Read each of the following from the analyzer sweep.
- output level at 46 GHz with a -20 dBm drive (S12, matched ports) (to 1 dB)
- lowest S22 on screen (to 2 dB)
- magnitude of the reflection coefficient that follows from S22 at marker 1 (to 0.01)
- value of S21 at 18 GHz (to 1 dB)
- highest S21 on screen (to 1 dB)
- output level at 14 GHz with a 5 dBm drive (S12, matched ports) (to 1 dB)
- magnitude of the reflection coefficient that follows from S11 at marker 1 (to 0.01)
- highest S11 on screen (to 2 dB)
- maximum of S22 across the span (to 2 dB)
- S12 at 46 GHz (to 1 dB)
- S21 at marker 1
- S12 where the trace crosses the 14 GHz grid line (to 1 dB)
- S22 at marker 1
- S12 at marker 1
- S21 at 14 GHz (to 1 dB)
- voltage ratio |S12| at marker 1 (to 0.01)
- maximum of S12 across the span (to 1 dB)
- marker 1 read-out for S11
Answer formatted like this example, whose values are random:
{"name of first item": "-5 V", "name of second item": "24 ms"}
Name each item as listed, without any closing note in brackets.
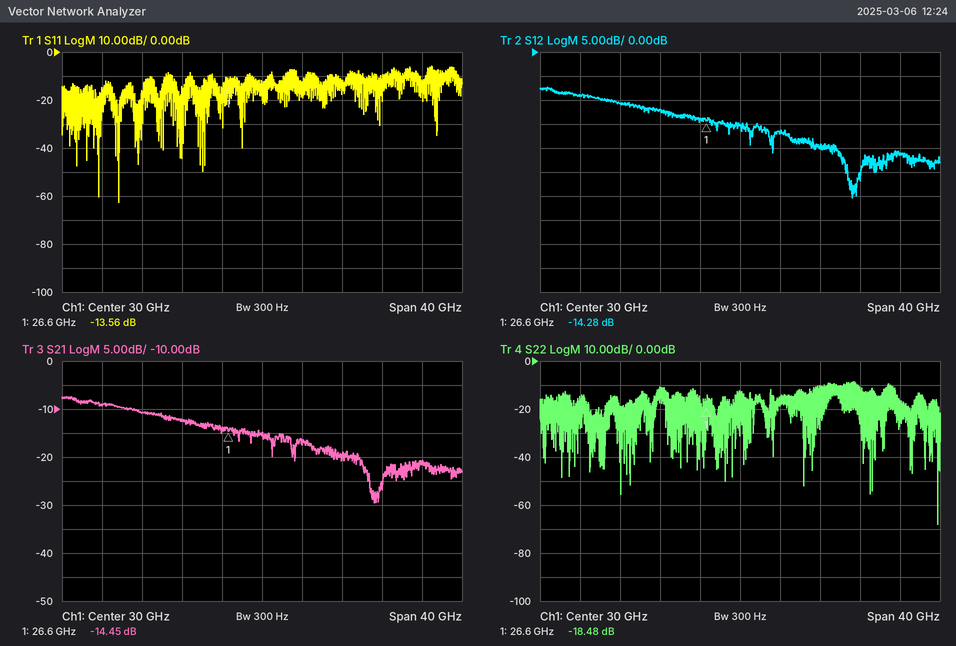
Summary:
{"output level at 46 GHz with a -20 dBm drive (S12, matched ports)": "-41 dBm", "lowest S22 on screen": "-68 dB", "magnitude of the reflection coefficient that follows from S22 at marker 1": "0.12", "value of S21 at 18 GHz": "-11 dB", "highest S21 on screen": "-7 dB", "output level at 14 GHz with a 5 dBm drive (S12, matched ports)": "-4 dBm", "magnitude of the reflection coefficient that follows from S11 at marker 1": "0.21", "highest S11 on screen": "-6 dB", "maximum of S22 across the span": "-8 dB", "S12 at 46 GHz": "-21 dB", "S21 at marker 1": "-14.45 dB", "S12 where the trace crosses the 14 GHz grid line": "-9 dB", "S22 at marker 1": "-18.48 dB", "S12 at marker 1": "-14.28 dB", "S21 at 14 GHz": "-9 dB", "voltage ratio |S12| at marker 1": "0.19", "maximum of S12 across the span": "-7 dB", "marker 1 read-out for S11": "-13.56 dB"}
